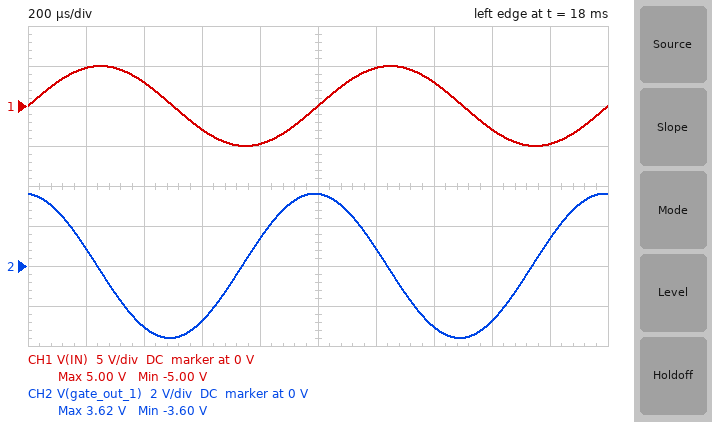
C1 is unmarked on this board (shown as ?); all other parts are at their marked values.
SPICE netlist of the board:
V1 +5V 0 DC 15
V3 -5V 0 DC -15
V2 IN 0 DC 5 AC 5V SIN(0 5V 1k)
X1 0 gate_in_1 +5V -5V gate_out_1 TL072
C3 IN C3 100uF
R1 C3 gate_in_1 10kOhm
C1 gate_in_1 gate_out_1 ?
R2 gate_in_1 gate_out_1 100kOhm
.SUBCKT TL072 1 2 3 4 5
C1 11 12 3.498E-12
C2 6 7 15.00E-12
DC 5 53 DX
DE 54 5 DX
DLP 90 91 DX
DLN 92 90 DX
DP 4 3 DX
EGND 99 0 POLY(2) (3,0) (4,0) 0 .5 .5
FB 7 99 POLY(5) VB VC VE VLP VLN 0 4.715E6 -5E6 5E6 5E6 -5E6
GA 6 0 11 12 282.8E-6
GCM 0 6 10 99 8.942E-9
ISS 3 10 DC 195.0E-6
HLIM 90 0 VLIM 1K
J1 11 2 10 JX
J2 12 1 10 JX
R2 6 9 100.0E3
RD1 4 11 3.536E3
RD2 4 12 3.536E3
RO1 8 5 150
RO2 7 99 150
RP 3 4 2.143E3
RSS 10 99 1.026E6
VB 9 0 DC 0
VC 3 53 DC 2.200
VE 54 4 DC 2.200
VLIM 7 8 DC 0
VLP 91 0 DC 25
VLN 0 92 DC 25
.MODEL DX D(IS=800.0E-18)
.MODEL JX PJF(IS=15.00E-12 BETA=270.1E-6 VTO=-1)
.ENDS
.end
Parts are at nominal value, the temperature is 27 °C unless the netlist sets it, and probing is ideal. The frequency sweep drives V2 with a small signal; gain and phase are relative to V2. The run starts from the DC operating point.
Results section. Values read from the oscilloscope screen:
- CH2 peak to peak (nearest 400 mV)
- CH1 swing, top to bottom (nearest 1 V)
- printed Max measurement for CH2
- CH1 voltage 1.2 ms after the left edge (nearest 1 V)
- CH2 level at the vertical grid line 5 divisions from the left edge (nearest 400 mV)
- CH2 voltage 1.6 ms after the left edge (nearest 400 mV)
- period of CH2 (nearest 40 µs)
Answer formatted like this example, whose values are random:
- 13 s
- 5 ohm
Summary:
- 7.2 V
- 10 V
- 3.62 V
- 5 V
- 3.6 V
- -2.8 V
- 1.00 ms
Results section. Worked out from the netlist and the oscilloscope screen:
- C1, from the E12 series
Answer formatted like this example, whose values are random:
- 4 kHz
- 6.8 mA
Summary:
- 22 nF
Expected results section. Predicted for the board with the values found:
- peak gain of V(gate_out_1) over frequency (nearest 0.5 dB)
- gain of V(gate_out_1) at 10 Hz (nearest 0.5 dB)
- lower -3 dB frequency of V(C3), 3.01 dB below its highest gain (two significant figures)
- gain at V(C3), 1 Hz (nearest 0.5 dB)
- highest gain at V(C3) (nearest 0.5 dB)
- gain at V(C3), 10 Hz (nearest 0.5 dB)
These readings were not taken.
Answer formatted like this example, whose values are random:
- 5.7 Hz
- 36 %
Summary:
- 20.0 dB
- 20.0 dB
- 160 mHz
- 0 dB
- 0 dB
- 0 dB
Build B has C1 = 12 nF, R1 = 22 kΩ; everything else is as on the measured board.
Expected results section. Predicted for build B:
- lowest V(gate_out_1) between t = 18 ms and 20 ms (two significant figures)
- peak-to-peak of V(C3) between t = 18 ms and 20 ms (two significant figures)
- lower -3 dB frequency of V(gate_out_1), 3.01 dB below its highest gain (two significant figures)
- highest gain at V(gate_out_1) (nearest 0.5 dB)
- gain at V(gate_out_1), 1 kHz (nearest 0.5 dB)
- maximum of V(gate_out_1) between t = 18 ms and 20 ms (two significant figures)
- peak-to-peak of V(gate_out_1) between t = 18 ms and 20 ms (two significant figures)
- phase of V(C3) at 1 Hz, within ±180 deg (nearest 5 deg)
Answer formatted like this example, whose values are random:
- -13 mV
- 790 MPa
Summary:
- -3.0 V
- 10 V
- 72 mHz
- 13.0 dB
- -4.5 dB
- 3.0 V
- 6.0 V
- 5 deg
